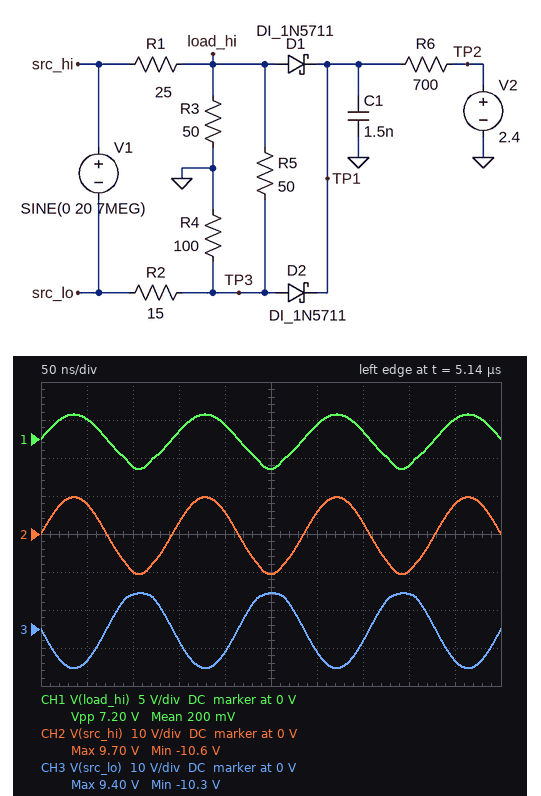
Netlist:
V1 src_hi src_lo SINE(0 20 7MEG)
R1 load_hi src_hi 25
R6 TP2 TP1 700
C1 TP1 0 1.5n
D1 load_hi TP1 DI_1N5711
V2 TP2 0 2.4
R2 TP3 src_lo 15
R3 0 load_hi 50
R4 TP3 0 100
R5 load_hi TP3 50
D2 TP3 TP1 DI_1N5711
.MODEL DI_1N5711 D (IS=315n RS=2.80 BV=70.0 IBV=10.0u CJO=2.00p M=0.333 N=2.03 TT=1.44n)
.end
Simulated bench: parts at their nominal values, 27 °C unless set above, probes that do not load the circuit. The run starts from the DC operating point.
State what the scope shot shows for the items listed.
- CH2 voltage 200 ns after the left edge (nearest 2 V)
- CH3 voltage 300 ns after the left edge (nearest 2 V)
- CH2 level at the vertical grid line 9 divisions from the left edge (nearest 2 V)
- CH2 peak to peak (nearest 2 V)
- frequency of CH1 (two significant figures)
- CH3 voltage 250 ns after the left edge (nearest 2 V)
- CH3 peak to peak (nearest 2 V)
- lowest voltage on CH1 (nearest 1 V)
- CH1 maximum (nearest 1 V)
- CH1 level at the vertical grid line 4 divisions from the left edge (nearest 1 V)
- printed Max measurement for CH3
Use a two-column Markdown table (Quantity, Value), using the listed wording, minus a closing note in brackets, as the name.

| Quantity | Value |
|---|---|
| CH2 voltage 200 ns after the left edge | 6 V |
| CH3 voltage 300 ns after the left edge | -6 V |
| CH2 level at the vertical grid line 9 divisions from the left edge | 8 V |
| CH2 peak to peak | 20 V |
| frequency of CH1 | 7.0 MHz |
| CH3 voltage 250 ns after the left edge | 10 V |
| CH3 peak to peak | 20 V |
| lowest voltage on CH1 | -4 V |
| CH1 maximum | 3 V |
| CH1 level at the vertical grid line 4 divisions from the left edge | 2 V |
| printed Max measurement for CH3 | 9.40 V |
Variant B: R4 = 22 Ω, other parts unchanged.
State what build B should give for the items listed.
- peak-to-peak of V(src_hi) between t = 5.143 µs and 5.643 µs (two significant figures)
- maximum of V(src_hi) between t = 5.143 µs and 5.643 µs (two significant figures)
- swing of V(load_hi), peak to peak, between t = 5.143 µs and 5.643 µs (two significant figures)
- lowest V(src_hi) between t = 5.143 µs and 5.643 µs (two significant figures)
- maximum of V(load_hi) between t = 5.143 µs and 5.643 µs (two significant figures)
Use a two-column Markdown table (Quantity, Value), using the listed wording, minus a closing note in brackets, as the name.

| Quantity | Value |
|---|---|
| peak-to-peak of V(src_hi) between t = 5.143 µs and 5.643 µs | 26 V |
| maximum of V(src_hi) between t = 5.143 µs and 5.643 µs | 13 V |
| swing of V(load_hi), peak to peak, between t = 5.143 µs and 5.643 µs | 11 V |
| lowest V(src_hi) between t = 5.143 µs and 5.643 µs | -13 V |
| maximum of V(load_hi) between t = 5.143 µs and 5.643 µs | 5.3 V |
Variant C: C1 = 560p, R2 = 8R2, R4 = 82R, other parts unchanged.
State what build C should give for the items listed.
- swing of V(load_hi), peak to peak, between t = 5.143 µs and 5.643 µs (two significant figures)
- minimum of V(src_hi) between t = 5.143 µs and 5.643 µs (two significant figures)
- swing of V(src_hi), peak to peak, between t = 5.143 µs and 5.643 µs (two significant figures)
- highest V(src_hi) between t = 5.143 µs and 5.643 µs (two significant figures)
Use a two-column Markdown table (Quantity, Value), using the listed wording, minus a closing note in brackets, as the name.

| Quantity | Value |
|---|---|
| swing of V(load_hi), peak to peak, between t = 5.143 µs and 5.643 µs | 8.6 V |
| minimum of V(src_hi) between t = 5.143 µs and 5.643 µs | -12 V |
| swing of V(src_hi), peak to peak, between t = 5.143 µs and 5.643 µs | 23 V |
| highest V(src_hi) between t = 5.143 µs and 5.643 µs | 11 V |
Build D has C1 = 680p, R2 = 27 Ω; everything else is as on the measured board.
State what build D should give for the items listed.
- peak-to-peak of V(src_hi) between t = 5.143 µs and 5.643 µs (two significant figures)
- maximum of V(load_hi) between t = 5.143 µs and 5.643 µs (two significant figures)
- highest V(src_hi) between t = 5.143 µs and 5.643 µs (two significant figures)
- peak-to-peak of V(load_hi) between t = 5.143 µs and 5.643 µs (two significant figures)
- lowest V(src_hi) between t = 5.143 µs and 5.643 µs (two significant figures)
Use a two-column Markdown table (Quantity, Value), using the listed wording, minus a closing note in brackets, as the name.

| Quantity | Value |
|---|---|
| peak-to-peak of V(src_hi) between t = 5.143 µs and 5.643 µs | 17 V |
| maximum of V(load_hi) between t = 5.143 µs and 5.643 µs | 2.8 V |
| highest V(src_hi) between t = 5.143 µs and 5.643 µs | 8.4 V |
| peak-to-peak of V(load_hi) between t = 5.143 µs and 5.643 µs | 6.1 V |
| lowest V(src_hi) between t = 5.143 µs and 5.643 µs | -9.0 V |
